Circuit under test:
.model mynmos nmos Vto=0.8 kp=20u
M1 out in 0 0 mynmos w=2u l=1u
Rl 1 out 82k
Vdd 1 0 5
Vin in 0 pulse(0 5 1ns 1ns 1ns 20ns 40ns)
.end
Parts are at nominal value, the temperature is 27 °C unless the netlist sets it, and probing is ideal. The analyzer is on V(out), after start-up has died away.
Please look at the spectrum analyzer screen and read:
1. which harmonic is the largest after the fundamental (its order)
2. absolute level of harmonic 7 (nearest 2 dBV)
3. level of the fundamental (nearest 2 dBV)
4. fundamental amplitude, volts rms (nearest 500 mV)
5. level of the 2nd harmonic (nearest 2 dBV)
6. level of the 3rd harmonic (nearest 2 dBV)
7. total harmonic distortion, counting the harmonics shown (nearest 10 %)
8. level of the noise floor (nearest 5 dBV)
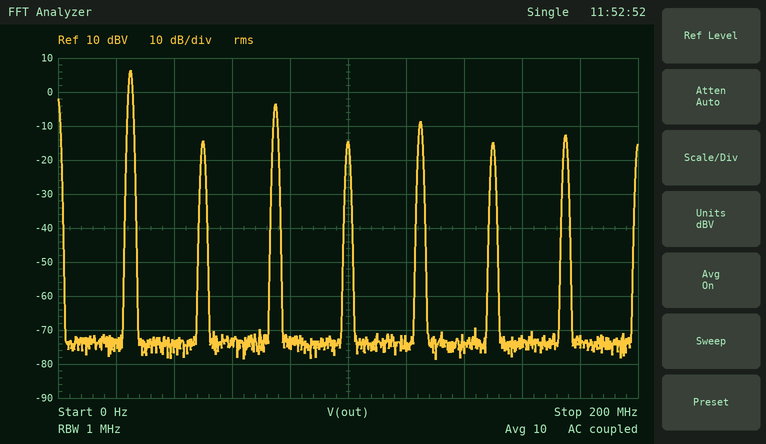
3
-12 dBV
6 dBV
2.0 V
-14 dBV
-4 dBV
40 %
-75 dBV
